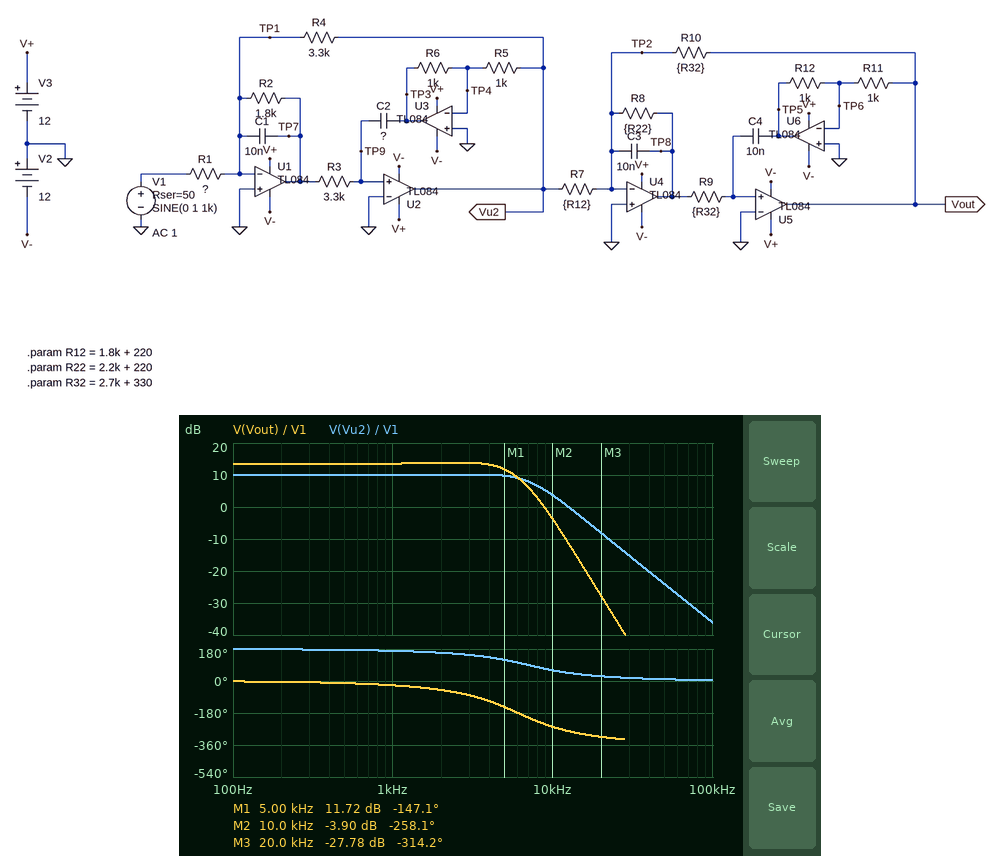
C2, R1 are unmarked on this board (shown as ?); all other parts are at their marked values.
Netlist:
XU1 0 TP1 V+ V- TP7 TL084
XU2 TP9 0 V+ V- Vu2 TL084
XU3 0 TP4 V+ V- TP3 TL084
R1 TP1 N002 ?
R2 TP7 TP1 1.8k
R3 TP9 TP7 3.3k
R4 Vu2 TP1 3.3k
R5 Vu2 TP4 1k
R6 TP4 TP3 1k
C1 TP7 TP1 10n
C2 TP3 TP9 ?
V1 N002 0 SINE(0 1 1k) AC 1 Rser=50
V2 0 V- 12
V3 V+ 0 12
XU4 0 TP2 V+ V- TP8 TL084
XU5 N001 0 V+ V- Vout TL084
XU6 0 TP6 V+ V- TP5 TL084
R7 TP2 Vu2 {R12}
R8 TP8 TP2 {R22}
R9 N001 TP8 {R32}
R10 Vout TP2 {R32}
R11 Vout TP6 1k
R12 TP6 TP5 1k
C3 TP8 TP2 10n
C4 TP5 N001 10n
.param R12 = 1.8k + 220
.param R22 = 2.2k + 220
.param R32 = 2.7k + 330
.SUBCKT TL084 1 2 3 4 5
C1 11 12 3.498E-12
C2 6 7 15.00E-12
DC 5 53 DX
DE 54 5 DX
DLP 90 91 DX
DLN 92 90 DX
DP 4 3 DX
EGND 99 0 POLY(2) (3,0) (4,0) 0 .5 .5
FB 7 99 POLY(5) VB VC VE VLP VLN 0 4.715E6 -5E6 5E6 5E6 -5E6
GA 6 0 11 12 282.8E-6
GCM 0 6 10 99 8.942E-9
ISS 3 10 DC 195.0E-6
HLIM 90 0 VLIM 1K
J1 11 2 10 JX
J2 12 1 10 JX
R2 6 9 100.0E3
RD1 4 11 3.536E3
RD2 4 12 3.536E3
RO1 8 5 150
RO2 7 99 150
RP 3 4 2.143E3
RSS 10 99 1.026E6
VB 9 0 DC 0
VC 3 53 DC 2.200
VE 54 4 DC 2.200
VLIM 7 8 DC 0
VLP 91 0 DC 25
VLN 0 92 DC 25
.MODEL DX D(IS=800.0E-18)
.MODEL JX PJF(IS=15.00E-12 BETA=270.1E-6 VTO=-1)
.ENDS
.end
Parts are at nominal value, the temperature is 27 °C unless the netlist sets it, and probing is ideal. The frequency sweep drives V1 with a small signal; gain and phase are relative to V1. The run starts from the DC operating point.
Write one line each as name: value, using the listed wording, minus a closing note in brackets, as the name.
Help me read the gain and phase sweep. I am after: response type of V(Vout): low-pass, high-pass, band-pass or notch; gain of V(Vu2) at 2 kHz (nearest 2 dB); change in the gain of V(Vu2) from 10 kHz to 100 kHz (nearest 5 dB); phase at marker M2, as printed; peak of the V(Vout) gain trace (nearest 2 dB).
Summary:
response type of V(Vout): low-pass, high-pass, band-pass or notch: low-pass
gain of V(Vu2) at 2 kHz: 10 dB
change in the gain of V(Vu2) from 10 kHz to 100 kHz: -40 dB
phase at marker M2, as printed: -258.1 deg
peak of the V(Vout) gain trace: 14 dB
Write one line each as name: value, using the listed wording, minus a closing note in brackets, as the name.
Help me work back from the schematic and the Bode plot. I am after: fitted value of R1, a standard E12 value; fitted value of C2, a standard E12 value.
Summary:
fitted value of R1, a standard E12 value: 1 kΩ
fitted value of C2, a standard E12 value: 4.7 nF
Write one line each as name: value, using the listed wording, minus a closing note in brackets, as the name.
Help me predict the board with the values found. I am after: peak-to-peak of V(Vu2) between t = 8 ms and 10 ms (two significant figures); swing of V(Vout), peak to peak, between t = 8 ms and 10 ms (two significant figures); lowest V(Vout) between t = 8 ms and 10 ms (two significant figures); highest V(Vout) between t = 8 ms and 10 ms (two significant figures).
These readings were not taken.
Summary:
peak-to-peak of V(Vu2) between t = 8 ms and 10 ms: 6.3 V
swing of V(Vout), peak to peak, between t = 8 ms and 10 ms: 9.5 V
lowest V(Vout) between t = 8 ms and 10 ms: -4.8 V
highest V(Vout) between t = 8 ms and 10 ms: 4.8 V
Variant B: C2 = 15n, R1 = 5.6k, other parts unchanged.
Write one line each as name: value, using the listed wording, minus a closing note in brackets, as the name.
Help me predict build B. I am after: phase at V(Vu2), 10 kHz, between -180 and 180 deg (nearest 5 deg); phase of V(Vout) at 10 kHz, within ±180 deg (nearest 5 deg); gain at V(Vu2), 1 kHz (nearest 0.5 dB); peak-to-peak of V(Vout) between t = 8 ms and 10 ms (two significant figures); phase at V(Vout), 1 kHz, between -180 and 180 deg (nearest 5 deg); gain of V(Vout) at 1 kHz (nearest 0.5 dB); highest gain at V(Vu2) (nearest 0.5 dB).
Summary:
phase at V(Vu2), 10 kHz, between -180 and 180 deg: 45 deg
phase of V(Vout) at 10 kHz, within ±180 deg: 90 deg
gain at V(Vu2), 1 kHz: -5.5 dB
peak-to-peak of V(Vout) between t = 8 ms and 10 ms: 1.6 V
phase at V(Vout), 1 kHz, between -180 and 180 deg: -45 deg
gain of V(Vout) at 1 kHz: -2.0 dB
highest gain at V(Vu2): -4.5 dB
